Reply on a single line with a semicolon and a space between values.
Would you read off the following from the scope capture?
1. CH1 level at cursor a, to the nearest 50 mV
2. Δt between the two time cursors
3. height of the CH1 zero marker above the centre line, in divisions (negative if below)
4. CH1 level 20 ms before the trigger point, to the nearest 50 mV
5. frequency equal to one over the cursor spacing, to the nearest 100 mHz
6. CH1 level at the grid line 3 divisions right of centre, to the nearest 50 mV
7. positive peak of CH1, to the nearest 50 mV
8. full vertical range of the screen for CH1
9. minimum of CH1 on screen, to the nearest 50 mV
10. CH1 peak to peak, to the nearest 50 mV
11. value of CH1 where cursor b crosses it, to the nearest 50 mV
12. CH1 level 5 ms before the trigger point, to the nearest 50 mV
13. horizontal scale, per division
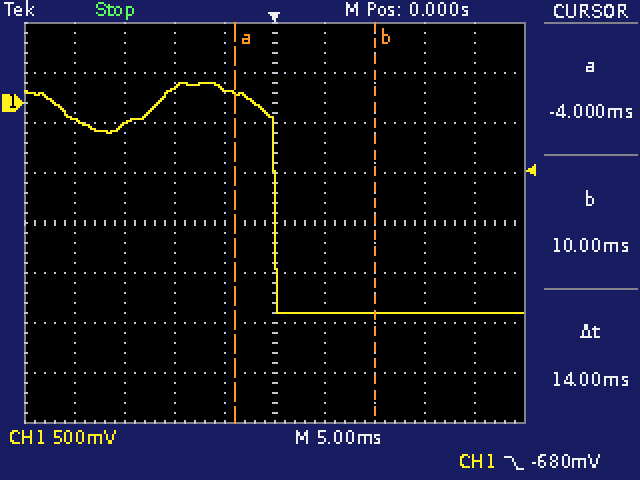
100 mV; 14 ms; +2.4 div; -150 mV; 71.4 Hz; -2.10 V; 200 mV; 4 V; -2.10 V; 2.30 V; -2.10 V; 150 mV; 5 ms
